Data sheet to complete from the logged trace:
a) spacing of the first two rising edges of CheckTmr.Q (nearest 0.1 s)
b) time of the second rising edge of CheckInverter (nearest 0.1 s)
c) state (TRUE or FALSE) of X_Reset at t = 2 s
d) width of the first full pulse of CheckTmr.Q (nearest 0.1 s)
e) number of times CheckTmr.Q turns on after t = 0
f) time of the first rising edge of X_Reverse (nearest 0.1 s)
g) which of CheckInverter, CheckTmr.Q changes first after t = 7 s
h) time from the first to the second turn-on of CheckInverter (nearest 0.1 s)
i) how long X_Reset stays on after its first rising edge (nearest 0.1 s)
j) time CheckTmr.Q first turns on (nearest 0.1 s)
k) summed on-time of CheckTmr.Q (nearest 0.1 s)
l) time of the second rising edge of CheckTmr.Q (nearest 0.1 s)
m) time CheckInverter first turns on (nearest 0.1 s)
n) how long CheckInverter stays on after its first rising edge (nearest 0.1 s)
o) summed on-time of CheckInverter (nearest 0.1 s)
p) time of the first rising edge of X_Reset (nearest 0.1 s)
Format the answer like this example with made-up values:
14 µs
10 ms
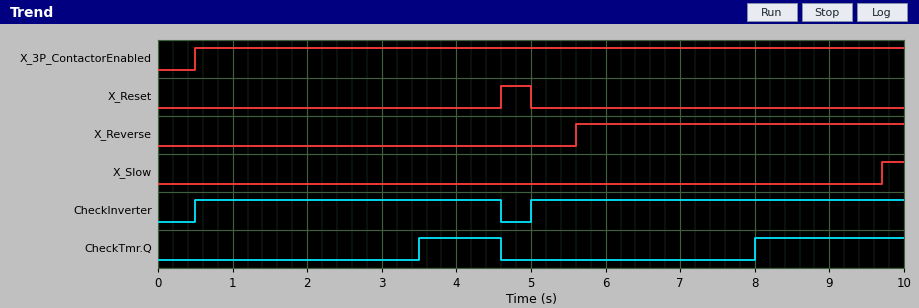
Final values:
4.5 s
5.0 s
FALSE
1.1 s
2
5.6 s
CheckTmr.Q
4.5 s
0.4 s
3.5 s
3.1 s
8.0 s
0.5 s
4.1 s
9.1 s
4.6 s
